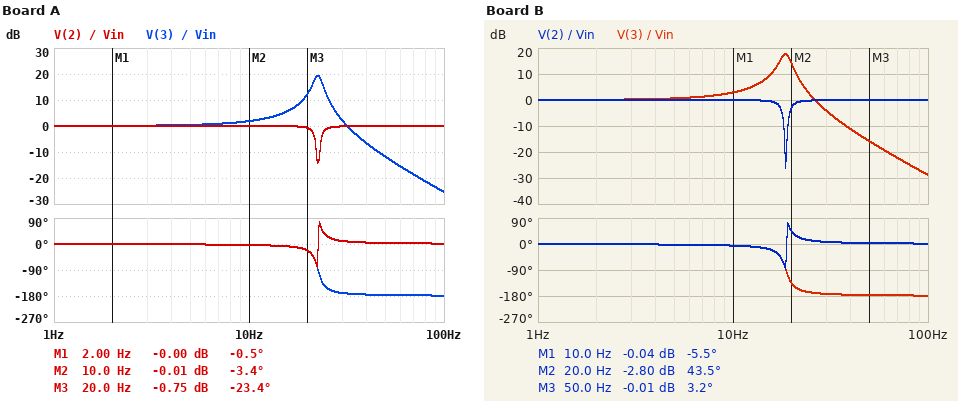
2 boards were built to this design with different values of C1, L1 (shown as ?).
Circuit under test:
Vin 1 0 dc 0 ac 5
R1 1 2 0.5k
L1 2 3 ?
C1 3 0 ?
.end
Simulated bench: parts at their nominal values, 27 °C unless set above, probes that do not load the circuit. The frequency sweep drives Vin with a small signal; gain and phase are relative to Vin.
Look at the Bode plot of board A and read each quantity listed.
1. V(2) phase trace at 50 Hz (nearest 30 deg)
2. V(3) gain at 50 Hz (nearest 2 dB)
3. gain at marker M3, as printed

0 deg
-12 dB
-0.75 dB
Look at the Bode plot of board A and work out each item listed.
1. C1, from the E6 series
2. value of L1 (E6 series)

1.5 µF
33 H
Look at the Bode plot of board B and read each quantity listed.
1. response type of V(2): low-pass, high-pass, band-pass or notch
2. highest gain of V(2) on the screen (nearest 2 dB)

notch
0 dB
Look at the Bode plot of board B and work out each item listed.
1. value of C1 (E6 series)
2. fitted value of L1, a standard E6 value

2.2 µF
33 H
